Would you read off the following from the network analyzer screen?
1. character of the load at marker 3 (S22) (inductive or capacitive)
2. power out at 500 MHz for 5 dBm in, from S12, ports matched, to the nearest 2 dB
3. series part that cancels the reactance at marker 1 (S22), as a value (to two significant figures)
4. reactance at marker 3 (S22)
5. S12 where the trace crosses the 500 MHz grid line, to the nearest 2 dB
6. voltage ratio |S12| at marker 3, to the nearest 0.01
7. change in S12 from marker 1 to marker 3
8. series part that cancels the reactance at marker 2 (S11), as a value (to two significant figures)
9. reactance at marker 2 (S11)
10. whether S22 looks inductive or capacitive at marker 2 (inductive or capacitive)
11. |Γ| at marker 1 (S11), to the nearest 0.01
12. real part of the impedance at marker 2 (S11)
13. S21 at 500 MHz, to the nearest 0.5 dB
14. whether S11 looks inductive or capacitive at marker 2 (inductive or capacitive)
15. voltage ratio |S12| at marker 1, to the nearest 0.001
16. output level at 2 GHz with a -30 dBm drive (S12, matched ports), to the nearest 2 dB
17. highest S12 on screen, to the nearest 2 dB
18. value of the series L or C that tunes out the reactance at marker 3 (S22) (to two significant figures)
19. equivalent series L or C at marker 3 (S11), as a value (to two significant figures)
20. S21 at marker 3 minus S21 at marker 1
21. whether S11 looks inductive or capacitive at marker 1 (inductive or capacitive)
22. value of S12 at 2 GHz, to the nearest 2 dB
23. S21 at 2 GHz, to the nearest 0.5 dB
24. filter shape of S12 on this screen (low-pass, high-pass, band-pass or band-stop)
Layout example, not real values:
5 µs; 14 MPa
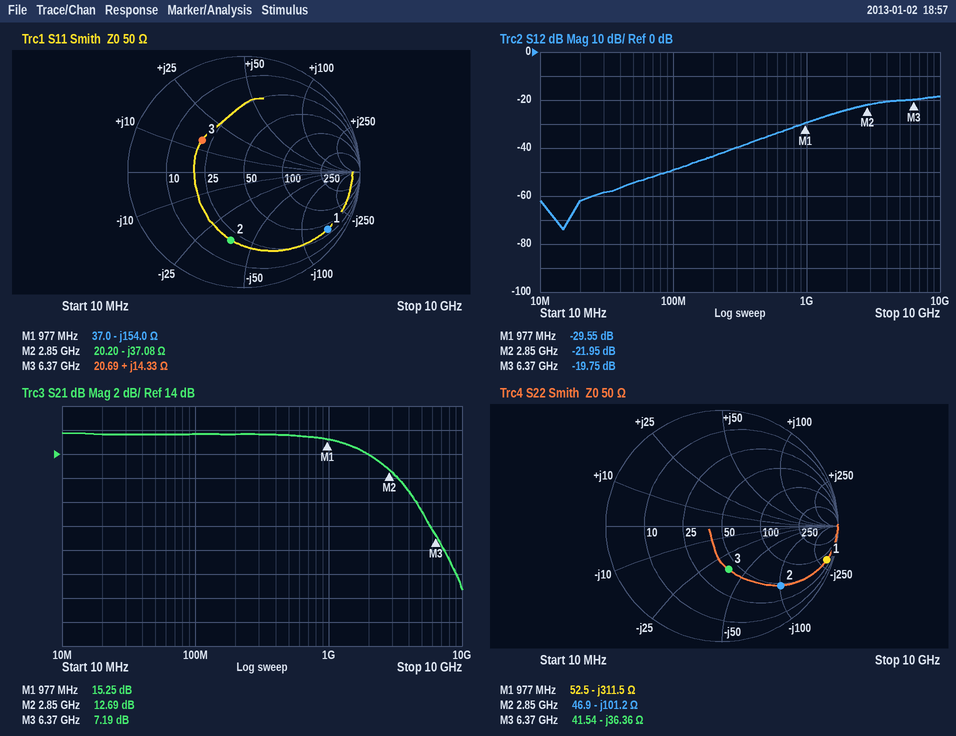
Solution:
capacitive; -30 dBm; 51 nH; -36.36 Ω; -36 dB; 0.10; 9.80 dB; 2.1 nH; -37.08 Ω; capacitive; 0.87; 20.20 Ω; 15.5 dB; capacitive; 0.033; -54 dBm; -18 dB; 910 pH; 360 pH; -8.06 dB; capacitive; -24 dB; 14.0 dB; high-pass
